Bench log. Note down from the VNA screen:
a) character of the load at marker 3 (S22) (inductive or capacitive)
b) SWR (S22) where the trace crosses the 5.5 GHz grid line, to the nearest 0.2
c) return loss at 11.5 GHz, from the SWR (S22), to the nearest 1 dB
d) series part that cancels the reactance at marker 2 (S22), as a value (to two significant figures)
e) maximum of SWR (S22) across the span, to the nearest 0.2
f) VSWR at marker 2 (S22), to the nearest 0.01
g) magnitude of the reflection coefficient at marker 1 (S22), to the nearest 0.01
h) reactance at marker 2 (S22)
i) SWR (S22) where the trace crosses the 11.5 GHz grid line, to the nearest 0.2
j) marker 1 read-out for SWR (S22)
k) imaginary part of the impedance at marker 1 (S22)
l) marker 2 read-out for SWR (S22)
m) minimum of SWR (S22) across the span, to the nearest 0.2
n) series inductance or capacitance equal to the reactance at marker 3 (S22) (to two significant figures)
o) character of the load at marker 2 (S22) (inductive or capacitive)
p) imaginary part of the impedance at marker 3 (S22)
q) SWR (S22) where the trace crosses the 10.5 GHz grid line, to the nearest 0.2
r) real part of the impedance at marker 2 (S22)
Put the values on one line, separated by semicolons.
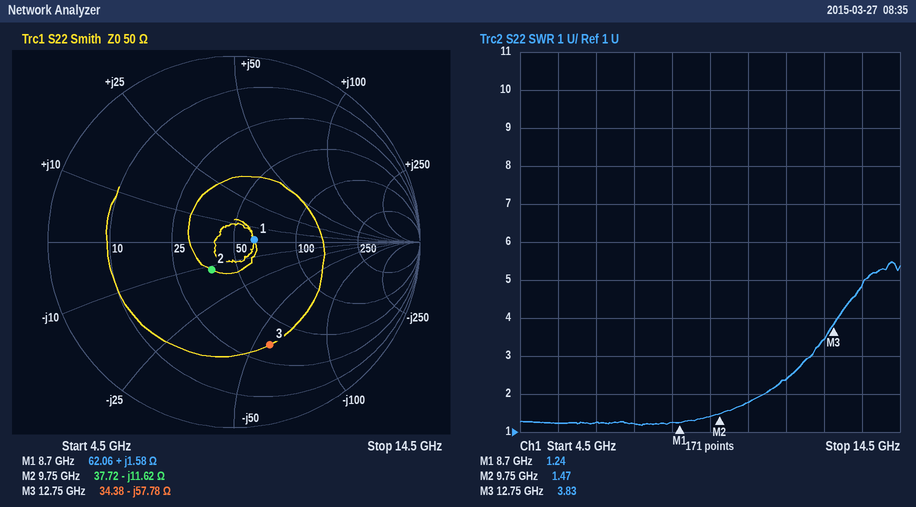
capacitive; 1.2; 8 dB; 190 pH; 5.4; 1.47; 0.11; -11.62 Ω; 2.4; 1.24; +1.58 Ω; 1.47; 1.2; 220 fF; capacitive; -57.78 Ω; 1.8; 37.72 Ω
